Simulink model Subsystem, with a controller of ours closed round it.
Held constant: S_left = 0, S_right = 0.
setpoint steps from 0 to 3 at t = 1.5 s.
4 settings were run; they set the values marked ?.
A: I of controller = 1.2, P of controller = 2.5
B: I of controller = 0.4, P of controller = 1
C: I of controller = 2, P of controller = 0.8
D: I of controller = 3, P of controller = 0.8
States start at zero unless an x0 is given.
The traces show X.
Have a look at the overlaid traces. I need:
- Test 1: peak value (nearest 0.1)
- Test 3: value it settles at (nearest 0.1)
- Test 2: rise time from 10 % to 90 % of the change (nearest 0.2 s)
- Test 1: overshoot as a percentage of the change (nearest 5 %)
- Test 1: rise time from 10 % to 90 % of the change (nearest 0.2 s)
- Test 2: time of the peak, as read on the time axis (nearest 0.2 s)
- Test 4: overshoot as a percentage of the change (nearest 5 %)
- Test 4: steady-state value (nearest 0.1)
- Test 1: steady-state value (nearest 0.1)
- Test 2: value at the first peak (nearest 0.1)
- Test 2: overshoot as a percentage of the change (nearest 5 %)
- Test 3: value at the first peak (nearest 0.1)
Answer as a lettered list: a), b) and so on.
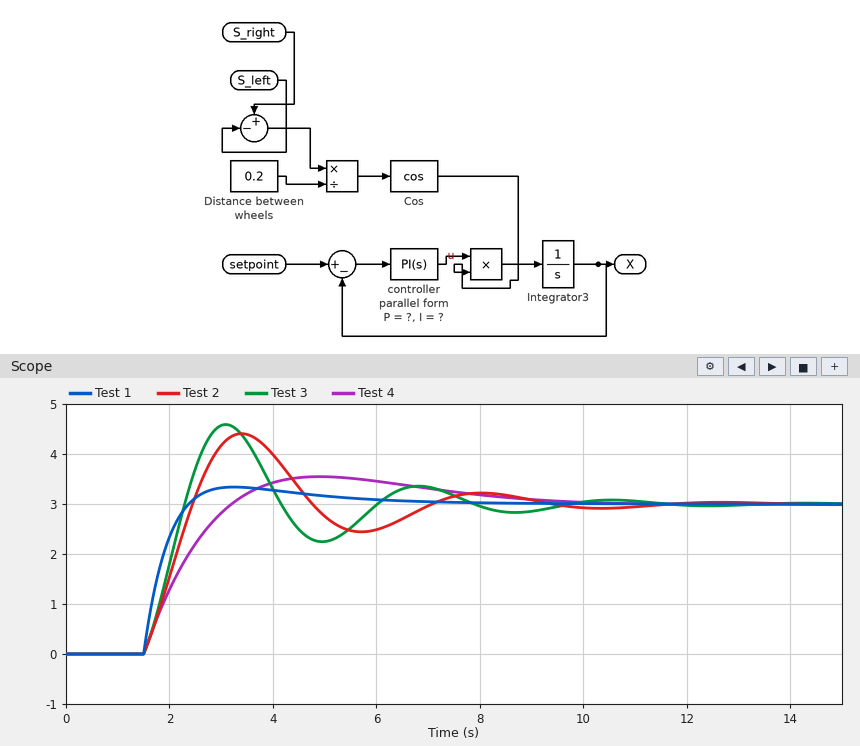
a) 3.3
b) 3.0
c) 0.8 s
d) 10 %
e) 0.6 s
f) 3.4 s
g) 20 %
h) 3.0
i) 3.0
j) 4.4
k) 45 %
l) 4.6
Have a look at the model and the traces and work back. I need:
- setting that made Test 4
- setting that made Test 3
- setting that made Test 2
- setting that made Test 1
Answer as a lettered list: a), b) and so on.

a) B
b) D
c) C
d) A
